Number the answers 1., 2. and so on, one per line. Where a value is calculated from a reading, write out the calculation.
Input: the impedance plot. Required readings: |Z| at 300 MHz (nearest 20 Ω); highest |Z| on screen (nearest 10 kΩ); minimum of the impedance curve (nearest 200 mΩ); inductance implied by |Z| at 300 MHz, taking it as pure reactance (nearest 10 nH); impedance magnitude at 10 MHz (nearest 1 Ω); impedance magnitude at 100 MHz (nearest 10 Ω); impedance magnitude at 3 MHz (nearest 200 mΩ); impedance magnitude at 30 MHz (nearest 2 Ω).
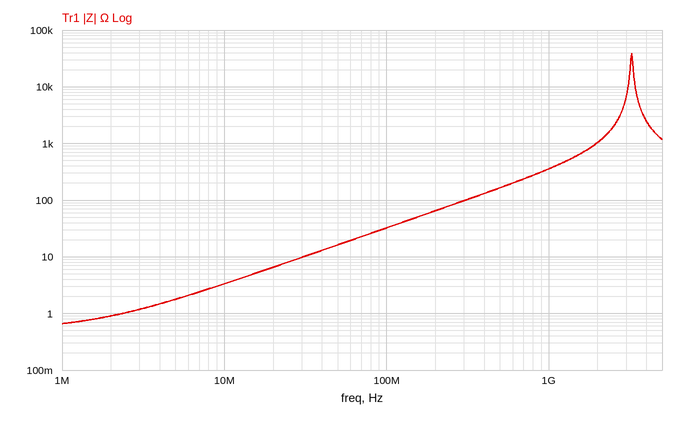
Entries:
1. 100 Ω
2. 40 kΩ
3. 600 mΩ
4. L = 100 Ω/(2π × 300 MHz) ≈ 53.1 nH, so 50 nH to the nearest 10 nH
5. 3 Ω
6. 30 Ω
7. 1.2 Ω
8. 10 Ω
